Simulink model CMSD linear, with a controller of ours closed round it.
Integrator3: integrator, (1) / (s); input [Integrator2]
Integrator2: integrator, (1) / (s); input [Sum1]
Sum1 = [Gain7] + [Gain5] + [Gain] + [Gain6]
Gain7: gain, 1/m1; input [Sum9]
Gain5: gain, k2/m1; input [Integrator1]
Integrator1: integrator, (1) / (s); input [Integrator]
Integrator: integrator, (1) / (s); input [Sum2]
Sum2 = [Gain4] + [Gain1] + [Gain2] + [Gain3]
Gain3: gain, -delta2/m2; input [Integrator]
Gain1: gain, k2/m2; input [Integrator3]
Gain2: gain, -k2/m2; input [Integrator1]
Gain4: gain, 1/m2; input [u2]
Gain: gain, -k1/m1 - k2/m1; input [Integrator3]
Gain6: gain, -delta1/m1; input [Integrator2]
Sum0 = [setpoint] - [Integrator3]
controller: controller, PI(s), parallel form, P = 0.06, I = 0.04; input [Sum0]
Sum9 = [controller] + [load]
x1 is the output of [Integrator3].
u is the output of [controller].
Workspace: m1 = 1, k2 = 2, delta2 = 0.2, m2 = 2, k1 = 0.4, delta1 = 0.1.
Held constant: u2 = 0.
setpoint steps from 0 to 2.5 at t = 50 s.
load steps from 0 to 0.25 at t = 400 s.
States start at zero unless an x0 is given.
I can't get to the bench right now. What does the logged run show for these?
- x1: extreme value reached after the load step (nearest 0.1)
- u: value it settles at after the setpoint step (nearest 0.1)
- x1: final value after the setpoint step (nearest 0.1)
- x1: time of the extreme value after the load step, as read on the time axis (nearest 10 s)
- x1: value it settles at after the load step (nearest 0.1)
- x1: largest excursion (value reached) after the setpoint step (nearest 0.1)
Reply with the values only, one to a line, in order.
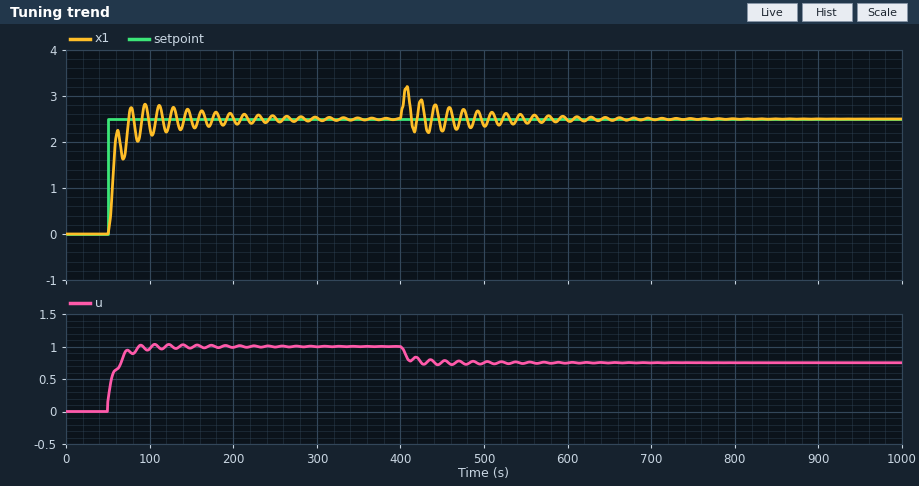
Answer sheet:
3.2
1.0
2.5
410 s
2.5
2.8
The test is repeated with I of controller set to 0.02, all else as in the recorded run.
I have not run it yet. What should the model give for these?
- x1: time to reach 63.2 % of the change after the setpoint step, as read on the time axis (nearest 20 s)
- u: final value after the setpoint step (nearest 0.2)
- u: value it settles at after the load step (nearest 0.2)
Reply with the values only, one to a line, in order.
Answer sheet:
80 s
1.0
0.8
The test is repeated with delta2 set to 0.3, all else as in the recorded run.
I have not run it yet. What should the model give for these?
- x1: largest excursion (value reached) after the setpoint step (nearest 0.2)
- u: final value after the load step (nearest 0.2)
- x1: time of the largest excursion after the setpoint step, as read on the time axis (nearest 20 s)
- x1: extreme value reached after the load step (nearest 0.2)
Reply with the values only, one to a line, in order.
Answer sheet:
2.6
0.8
100 s
3.2
